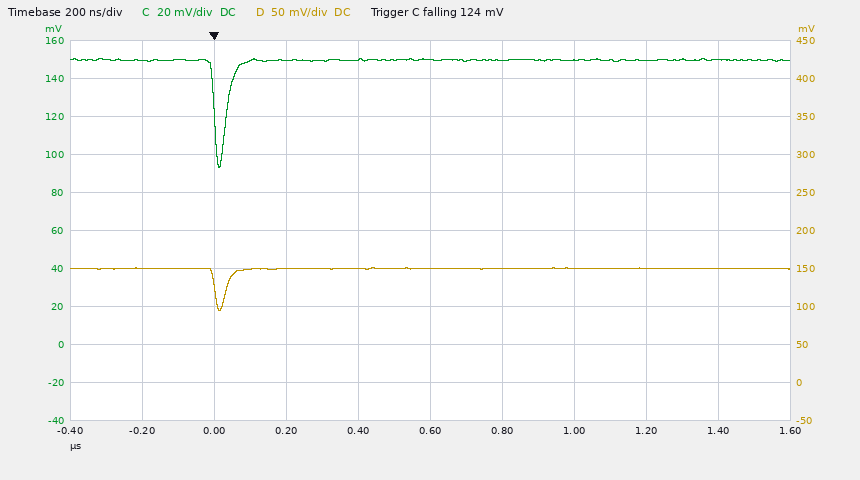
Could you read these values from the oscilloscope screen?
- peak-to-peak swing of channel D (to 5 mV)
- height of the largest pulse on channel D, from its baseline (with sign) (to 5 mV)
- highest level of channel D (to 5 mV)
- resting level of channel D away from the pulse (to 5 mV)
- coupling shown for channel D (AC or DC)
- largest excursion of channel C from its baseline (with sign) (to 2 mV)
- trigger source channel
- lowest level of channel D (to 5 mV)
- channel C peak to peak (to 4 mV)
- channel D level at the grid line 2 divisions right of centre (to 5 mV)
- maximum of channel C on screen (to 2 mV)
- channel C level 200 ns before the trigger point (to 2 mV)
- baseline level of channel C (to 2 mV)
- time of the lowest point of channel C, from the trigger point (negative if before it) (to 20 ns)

55 mV
-55 mV
150 mV
150 mV
DC
-56 mV
channel C
95 mV
56 mV
150 mV
150 mV
150 mV
150 mV
+20 ns
